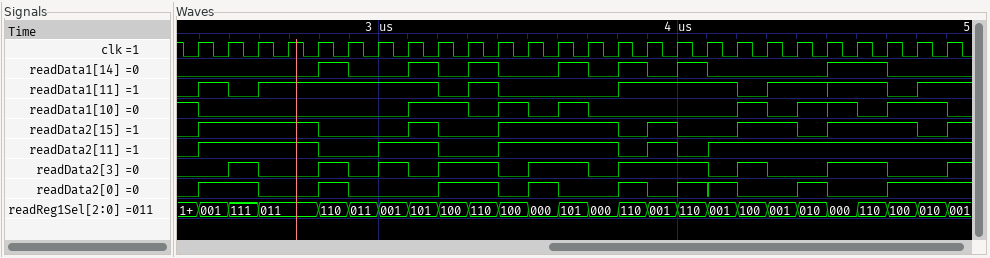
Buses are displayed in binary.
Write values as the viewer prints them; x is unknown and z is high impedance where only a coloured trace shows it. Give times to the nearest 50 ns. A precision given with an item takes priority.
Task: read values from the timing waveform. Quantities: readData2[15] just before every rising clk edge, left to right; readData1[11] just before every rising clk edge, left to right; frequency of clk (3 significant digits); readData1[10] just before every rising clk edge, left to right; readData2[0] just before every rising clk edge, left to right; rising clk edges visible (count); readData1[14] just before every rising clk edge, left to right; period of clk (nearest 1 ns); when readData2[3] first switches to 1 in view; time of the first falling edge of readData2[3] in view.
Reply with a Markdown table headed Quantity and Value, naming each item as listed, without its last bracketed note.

| Quantity | Value |
|---|---|
| readData2[15] just before every rising clk edge, left to right | 0 1 1 1 1 0 0 0 1 0 0 1 1 1 1 0 1 0 0 1 1 0 1 1 1 0 |
| readData1[11] just before every rising clk edge, left to right | 0 1 0 1 1 1 1 1 1 0 1 0 0 0 0 1 1 1 1 0 1 1 1 1 0 1 |
| frequency of clk | 10.0 MHz |
| readData1[10] just before every rising clk edge, left to right | 1 0 0 0 0 0 0 0 1 1 0 1 0 1 0 0 0 0 0 1 0 1 1 0 1 1 |
| readData2[0] just before every rising clk edge, left to right | 0 1 1 0 0 1 0 0 0 1 1 0 1 0 0 1 0 1 1 0 0 1 0 0 1 1 |
| rising clk edges visible | 26 |
| readData1[14] just before every rising clk edge, left to right | 0 0 0 0 0 1 0 0 1 0 1 0 0 1 0 1 0 1 0 0 0 0 1 1 0 0 |
| period of clk | 100 ns |
| when readData2[3] first switches to 1 in view | 2500 ns |
| time of the first falling edge of readData2[3] in view | 2600 ns |
